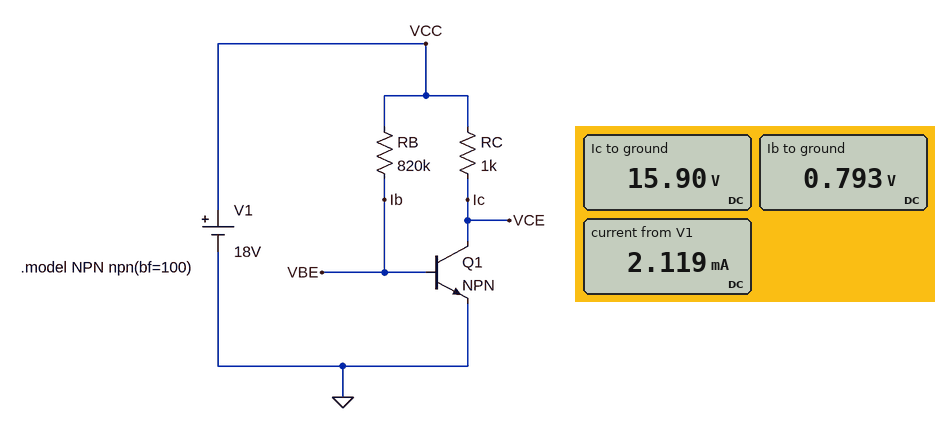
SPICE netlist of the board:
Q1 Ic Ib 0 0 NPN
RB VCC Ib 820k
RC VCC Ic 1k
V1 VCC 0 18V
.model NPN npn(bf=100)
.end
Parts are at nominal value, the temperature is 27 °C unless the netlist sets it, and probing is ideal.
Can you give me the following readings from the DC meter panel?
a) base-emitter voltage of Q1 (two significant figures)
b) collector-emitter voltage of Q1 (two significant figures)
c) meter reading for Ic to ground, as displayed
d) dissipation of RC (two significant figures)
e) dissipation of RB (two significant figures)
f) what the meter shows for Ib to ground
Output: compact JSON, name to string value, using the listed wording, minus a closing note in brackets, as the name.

{"base-emitter voltage of Q1": "790 mV", "collector-emitter voltage of Q1": "16 V", "meter reading for Ic to ground, as displayed": "15.90 V", "dissipation of RC": "4.4 mW", "dissipation of RB": "360 µW", "what the meter shows for Ib to ground": "0.793 V"}
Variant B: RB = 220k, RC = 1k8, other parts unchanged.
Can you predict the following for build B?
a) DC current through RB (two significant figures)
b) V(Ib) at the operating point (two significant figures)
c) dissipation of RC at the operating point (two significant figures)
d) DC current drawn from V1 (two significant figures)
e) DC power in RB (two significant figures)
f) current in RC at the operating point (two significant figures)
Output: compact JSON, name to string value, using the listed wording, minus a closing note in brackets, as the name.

{"DC current through RB": "78 µA", "V(Ib) at the operating point": "830 mV", "dissipation of RC at the operating point": "110 mW", "DC current drawn from V1": "7.9 mA", "DC power in RB": "1.3 mW", "current in RC at the operating point": "7.8 mA"}
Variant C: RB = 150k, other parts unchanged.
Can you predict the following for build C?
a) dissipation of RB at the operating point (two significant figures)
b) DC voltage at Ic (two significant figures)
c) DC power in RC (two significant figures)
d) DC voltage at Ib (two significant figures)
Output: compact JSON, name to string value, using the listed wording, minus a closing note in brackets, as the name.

{"dissipation of RB at the operating point": "2.0 mW", "DC voltage at Ic": "6.6 V", "DC power in RC": "130 mW", "DC voltage at Ib": "840 mV"}
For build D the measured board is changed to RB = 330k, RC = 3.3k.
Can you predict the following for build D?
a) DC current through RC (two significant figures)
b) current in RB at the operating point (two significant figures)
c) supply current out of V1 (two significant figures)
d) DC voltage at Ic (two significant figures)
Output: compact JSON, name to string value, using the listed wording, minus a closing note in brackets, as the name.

{"DC current through RC": "5.2 mA", "current in RB at the operating point": "52 µA", "supply current out of V1": "5.3 mA", "DC voltage at Ic": "820 mV"}
